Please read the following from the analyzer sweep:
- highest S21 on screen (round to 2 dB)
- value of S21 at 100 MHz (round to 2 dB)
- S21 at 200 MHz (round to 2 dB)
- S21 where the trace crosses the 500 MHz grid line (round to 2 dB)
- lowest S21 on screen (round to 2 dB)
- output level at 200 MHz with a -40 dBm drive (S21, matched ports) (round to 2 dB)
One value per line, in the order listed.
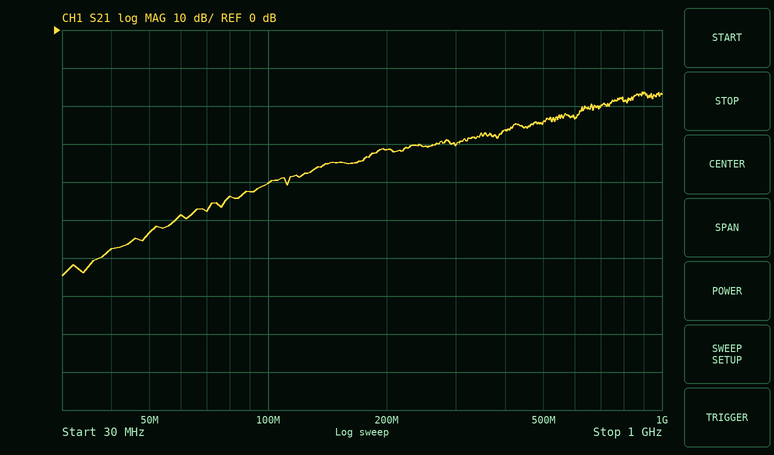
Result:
-16 dB
-40 dB
-32 dB
-24 dB
-64 dB
-72 dBm
